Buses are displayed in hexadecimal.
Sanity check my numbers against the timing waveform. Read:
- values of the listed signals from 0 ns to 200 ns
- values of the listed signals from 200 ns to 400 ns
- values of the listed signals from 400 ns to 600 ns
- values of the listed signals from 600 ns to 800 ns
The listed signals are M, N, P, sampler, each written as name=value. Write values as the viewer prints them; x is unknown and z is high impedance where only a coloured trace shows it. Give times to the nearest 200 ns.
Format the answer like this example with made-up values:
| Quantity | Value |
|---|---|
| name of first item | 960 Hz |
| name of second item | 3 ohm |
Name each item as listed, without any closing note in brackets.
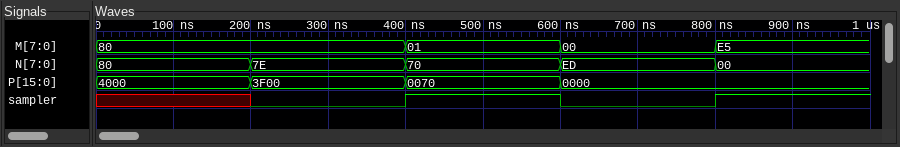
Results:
| Quantity | Value |
|---|---|
| values of the listed signals from 0 ns to 200 ns | M=80, N=80, P=4000, sampler=x |
| values of the listed signals from 200 ns to 400 ns | M=80, N=7E, P=3F00, sampler=0 |
| values of the listed signals from 400 ns to 600 ns | M=01, N=70, P=0070, sampler=1 |
| values of the listed signals from 600 ns to 800 ns | M=00, N=ED, P=0000, sampler=0 |
